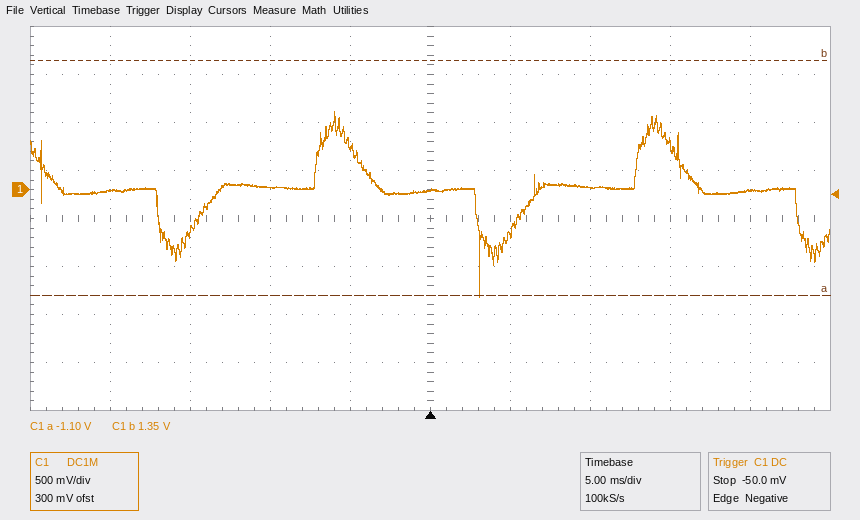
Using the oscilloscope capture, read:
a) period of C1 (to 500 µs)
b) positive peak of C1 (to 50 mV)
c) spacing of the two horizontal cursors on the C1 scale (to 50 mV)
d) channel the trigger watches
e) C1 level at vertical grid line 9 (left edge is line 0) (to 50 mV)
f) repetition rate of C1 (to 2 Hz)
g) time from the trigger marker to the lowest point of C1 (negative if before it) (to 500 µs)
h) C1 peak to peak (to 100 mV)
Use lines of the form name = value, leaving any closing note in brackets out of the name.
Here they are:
period of C1 = 20.0 ms
positive peak of C1 = 800 mV
spacing of the two horizontal cursors on the C1 scale = 2.45 V
channel the trigger watches = C1
C1 level at vertical grid line 9 (left edge is line 0) = 0 mV
repetition rate of C1 = 50 Hz
time from the trigger marker to the lowest point of C1 (negative if before it) = +3.0 ms
C1 peak to peak = 1.90 V
